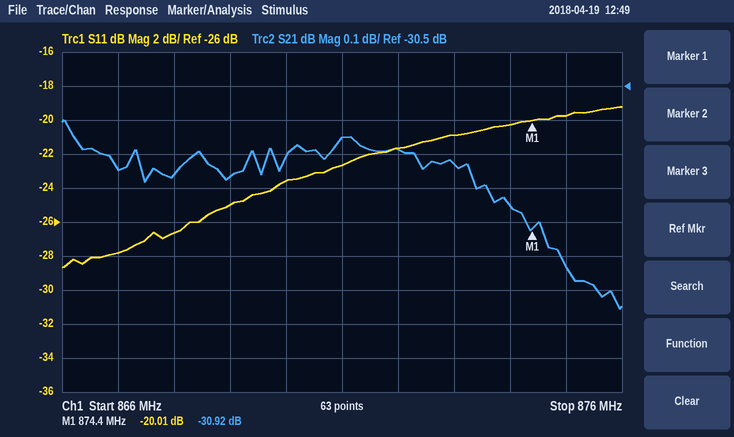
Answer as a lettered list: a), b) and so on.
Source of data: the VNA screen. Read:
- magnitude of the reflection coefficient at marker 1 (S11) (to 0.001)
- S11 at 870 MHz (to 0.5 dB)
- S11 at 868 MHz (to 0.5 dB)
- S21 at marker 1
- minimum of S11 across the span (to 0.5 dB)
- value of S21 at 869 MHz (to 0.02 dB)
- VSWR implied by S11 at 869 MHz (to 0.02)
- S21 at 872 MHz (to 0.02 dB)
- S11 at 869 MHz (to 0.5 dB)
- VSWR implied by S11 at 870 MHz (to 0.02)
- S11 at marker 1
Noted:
a) 0.100
b) -23.5 dB
c) -26.5 dB
d) -30.92 dB
e) -28.5 dB
f) -30.76 dB
g) 1.12
h) -30.68 dB
i) -25.0 dB
j) 1.14
k) -20.01 dB
